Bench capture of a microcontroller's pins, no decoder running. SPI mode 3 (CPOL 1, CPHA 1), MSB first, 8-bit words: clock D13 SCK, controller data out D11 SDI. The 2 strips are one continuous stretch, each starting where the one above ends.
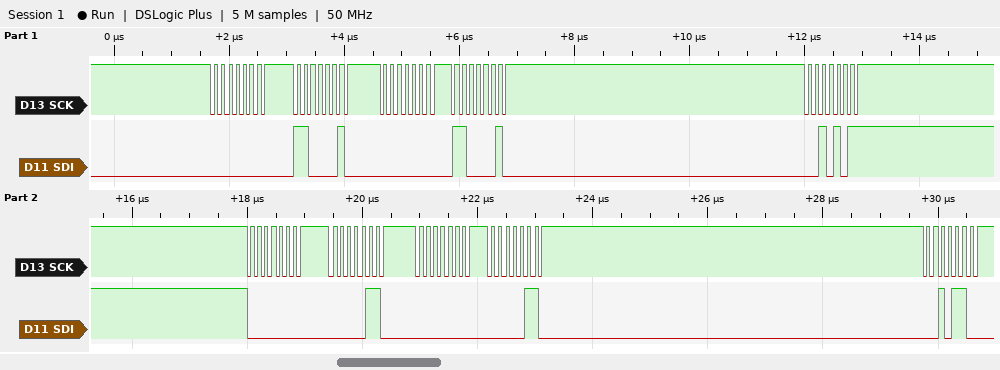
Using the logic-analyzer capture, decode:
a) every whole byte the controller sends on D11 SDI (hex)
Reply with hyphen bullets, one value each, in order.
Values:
- 00 C2 00 C2 2B 00 06 00 06 2C
